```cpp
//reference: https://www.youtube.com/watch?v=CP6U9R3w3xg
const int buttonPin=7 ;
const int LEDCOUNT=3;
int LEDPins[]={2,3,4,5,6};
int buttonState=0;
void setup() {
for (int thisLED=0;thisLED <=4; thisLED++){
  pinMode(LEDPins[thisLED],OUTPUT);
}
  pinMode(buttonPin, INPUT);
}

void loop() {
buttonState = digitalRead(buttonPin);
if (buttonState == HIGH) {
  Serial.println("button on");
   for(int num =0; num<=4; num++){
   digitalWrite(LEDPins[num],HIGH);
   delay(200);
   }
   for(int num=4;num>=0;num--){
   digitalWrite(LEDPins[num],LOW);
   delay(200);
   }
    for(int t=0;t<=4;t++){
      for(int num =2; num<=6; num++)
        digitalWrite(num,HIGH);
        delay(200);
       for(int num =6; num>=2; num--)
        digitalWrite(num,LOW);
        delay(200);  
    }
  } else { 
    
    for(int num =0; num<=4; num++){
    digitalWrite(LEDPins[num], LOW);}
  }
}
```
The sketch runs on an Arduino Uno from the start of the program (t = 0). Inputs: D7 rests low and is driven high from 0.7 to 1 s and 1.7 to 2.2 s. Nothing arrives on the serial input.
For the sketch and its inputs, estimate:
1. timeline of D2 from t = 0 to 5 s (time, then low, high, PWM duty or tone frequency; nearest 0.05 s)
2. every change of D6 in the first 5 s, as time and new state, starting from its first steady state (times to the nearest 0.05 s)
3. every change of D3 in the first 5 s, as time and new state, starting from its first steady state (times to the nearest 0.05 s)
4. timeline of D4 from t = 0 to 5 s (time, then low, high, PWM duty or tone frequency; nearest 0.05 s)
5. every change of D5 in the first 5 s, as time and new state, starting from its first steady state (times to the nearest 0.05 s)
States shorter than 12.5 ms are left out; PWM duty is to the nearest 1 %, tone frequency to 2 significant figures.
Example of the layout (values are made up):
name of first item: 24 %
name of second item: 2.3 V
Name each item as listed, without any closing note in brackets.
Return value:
timeline of D2 from t = 0 to 5 s: 0 s low; 0.7 s high; 2.5 s low; 2.7 s high; 2.9 s low; 3.1 s high; 3.3 s low; 3.5 s high; 3.7 s low; 3.9 s high; 4.1 s low; 4.3 s high; 4.5 s low
every change of D6 in the first 5 s, as time and new state, starting from its first steady state: 0 s low; 1.5 s high; 1.7 s low; 2.7 s high; 2.9 s low; 3.1 s high; 3.3 s low; 3.5 s high; 3.7 s low; 3.9 s high; 4.1 s low; 4.3 s high; 4.5 s low
every change of D3 in the first 5 s, as time and new state, starting from its first steady state: 0 s low; 0.9 s high; 2.3 s low; 2.7 s high; 2.9 s low; 3.1 s high; 3.3 s low; 3.5 s high; 3.7 s low; 3.9 s high; 4.1 s low; 4.3 s high; 4.5 s low
timeline of D4 from t = 0 to 5 s: 0 s low; 1.1 s high; 2.1 s low; 2.7 s high; 2.9 s low; 3.1 s high; 3.3 s low; 3.5 s high; 3.7 s low; 3.9 s high; 4.1 s low; 4.3 s high; 4.5 s low
every change of D5 in the first 5 s, as time and new state, starting from its first steady state: 0 s low; 1.3 s high; 1.9 s low; 2.7 s high; 2.9 s low; 3.1 s high; 3.3 s low; 3.5 s high; 3.7 s low; 3.9 s high; 4.1 s low; 4.3 s high; 4.5 s low
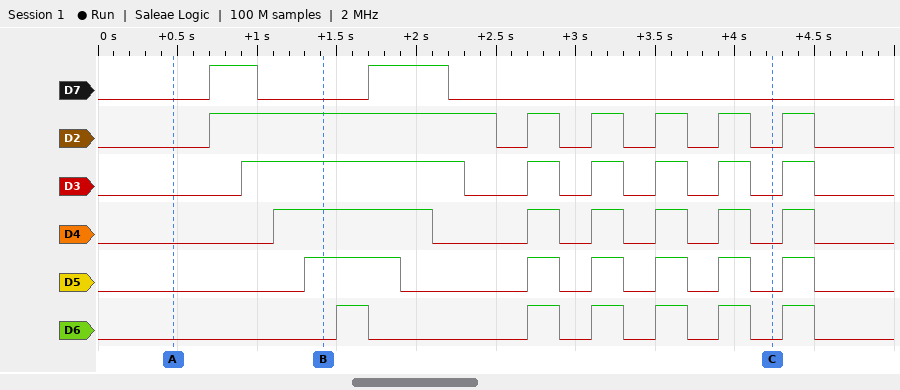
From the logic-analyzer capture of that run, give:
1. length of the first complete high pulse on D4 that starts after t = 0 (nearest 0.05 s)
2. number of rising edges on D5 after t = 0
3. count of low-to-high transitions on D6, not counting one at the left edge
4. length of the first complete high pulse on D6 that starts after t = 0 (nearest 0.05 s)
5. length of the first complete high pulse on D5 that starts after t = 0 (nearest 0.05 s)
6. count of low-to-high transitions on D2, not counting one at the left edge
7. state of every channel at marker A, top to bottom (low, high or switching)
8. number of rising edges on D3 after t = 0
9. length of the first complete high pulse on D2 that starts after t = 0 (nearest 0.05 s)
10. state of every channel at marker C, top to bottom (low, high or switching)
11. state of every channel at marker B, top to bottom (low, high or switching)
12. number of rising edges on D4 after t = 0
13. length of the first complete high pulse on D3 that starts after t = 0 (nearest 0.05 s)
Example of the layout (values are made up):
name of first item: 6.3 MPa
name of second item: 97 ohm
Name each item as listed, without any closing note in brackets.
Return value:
length of the first complete high pulse on D4 that starts after t = 0: 1.00 s
number of rising edges on D5 after t = 0: 6
count of low-to-high transitions on D6, not counting one at the left edge: 6
length of the first complete high pulse on D6 that starts after t = 0: 0.20 s
length of the first complete high pulse on D5 that starts after t = 0: 0.60 s
count of low-to-high transitions on D2, not counting one at the left edge: 6
state of every channel at marker A, top to bottom: D7 low, D2 low, D3 low, D4 low, D5 low, D6 low
number of rising edges on D3 after t = 0: 6
length of the first complete high pulse on D2 that starts after t = 0: 1.80 s
state of every channel at marker C, top to bottom: D7 low, D2 low, D3 low, D4 low, D5 low, D6 low
state of every channel at marker B, top to bottom: D7 low, D2 high, D3 high, D4 high, D5 high, D6 low
number of rising edges on D4 after t = 0: 6
length of the first complete high pulse on D3 that starts after t = 0: 1.40 s
